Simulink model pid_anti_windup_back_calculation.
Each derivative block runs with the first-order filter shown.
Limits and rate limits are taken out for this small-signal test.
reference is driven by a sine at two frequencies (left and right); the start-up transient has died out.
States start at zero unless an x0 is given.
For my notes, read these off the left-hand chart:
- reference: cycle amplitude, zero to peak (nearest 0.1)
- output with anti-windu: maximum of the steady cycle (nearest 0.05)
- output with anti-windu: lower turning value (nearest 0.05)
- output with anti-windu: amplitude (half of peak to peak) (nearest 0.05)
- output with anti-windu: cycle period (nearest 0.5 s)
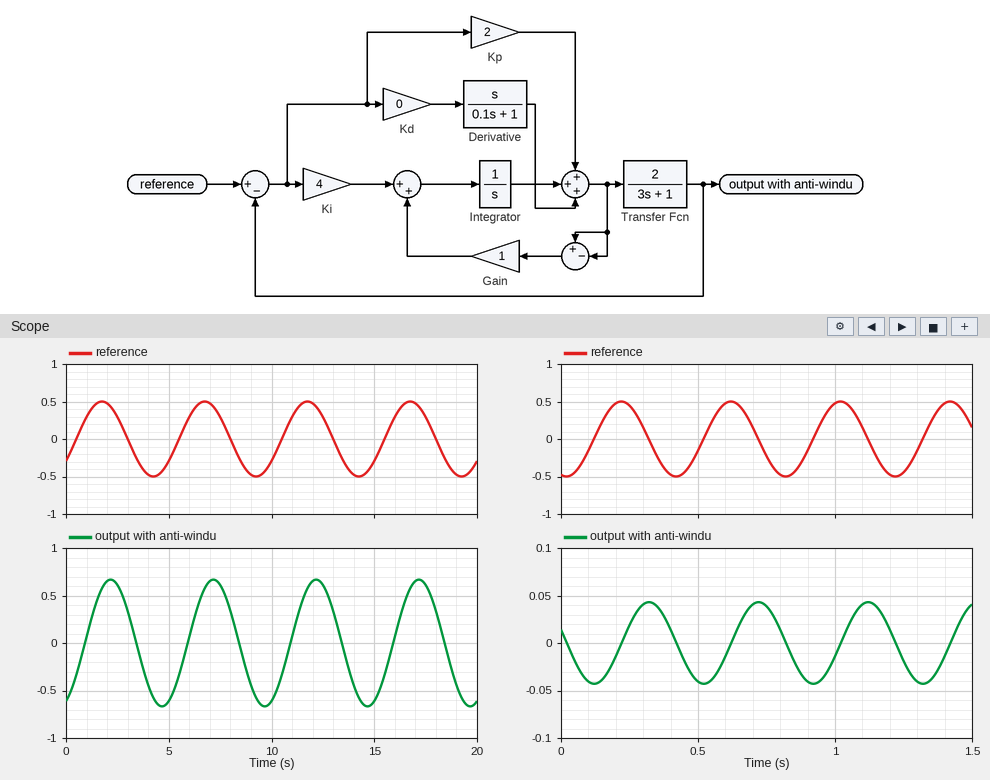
0.5
0.65
-0.65
0.65
5.0 s
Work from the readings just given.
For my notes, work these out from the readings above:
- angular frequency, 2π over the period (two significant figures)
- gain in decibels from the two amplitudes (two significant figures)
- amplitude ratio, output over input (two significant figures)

1.3 rad/s
2.3 dB
1.3
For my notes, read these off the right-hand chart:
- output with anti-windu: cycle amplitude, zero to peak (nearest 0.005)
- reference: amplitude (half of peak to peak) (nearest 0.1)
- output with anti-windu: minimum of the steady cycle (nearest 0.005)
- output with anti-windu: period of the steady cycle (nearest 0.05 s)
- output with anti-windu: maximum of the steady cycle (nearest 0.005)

0.045
0.5
-0.045
0.40 s
0.045
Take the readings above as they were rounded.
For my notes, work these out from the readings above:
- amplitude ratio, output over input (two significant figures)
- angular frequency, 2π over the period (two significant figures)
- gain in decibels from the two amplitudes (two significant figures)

0.090
16 rad/s
-21 dB
